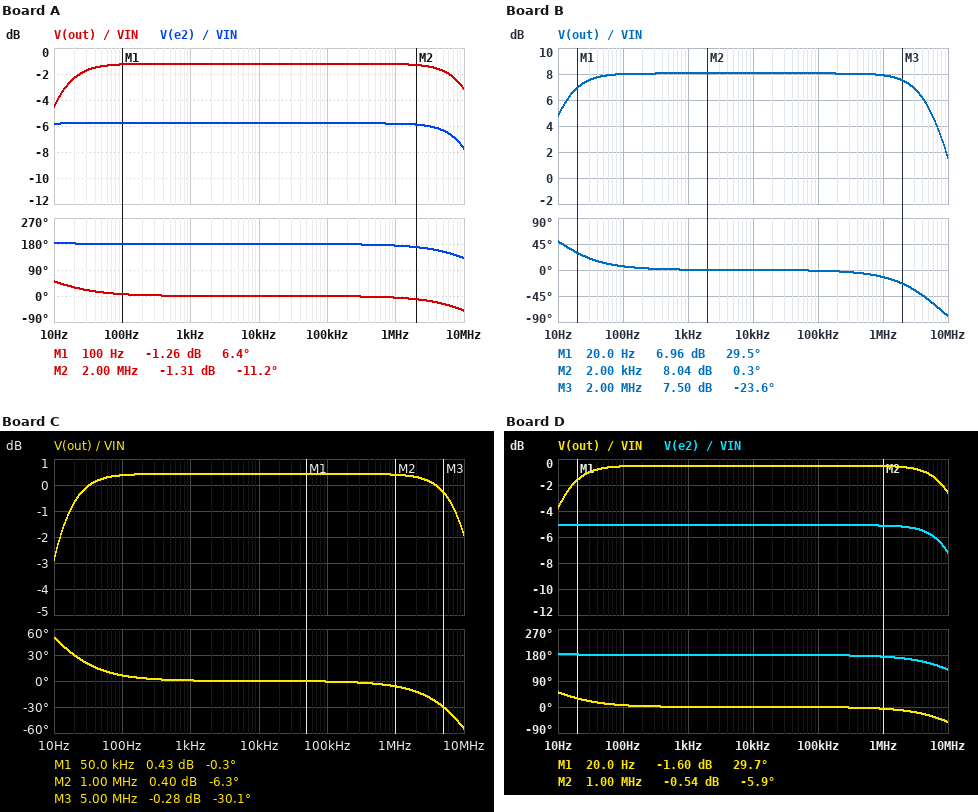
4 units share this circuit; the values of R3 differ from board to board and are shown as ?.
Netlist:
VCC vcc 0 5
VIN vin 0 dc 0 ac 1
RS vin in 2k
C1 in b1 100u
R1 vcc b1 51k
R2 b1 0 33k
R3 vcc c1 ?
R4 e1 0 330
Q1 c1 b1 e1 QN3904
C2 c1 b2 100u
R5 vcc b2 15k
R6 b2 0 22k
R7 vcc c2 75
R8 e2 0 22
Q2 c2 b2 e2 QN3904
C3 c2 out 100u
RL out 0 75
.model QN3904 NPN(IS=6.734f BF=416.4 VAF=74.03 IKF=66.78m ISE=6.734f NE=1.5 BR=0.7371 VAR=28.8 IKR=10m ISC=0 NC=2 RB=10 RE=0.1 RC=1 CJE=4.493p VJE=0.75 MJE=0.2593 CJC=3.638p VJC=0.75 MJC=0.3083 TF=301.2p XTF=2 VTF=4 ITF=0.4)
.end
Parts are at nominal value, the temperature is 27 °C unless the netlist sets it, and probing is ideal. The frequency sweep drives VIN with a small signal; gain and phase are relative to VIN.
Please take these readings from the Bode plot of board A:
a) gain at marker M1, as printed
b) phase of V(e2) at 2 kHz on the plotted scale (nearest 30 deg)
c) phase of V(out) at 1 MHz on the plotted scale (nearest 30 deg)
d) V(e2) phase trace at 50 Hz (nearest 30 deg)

-1.26 dB
180 deg
0 deg
180 deg
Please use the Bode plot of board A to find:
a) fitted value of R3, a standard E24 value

220 Ω
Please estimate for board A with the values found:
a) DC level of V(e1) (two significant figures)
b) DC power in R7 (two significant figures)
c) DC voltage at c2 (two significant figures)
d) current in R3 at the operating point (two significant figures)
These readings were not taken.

1.1 V
110 mW
2.1 V
3.3 mA
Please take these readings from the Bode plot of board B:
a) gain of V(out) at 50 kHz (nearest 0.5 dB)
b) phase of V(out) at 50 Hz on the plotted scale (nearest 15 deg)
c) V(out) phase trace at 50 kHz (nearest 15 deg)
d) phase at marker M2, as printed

8.0 dB
15 deg
0 deg
0.3 deg
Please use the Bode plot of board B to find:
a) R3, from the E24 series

750 Ω
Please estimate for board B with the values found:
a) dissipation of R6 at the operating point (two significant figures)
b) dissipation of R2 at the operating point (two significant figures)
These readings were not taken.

120 µW
97 µW
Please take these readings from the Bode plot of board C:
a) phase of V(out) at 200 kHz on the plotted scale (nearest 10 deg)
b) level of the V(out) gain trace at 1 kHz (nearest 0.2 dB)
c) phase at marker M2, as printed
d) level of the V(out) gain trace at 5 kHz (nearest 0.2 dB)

0 deg
0.4 dB
-6.3 deg
0.4 dB
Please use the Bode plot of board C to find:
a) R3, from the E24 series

270 Ω
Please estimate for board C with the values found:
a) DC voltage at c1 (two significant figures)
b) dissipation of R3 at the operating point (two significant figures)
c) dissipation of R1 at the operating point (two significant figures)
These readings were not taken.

4.1 V
2.9 mW
200 µW
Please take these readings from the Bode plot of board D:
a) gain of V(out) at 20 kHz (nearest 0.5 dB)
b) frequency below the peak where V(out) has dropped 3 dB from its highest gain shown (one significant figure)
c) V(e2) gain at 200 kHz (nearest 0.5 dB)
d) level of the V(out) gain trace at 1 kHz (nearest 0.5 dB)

-0.5 dB
10 Hz
-5.0 dB
-0.5 dB
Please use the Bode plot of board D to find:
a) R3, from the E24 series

240 Ω
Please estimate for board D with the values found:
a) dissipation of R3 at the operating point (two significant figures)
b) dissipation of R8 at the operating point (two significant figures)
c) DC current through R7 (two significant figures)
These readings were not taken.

2.6 mW
32 mW
38 mA
